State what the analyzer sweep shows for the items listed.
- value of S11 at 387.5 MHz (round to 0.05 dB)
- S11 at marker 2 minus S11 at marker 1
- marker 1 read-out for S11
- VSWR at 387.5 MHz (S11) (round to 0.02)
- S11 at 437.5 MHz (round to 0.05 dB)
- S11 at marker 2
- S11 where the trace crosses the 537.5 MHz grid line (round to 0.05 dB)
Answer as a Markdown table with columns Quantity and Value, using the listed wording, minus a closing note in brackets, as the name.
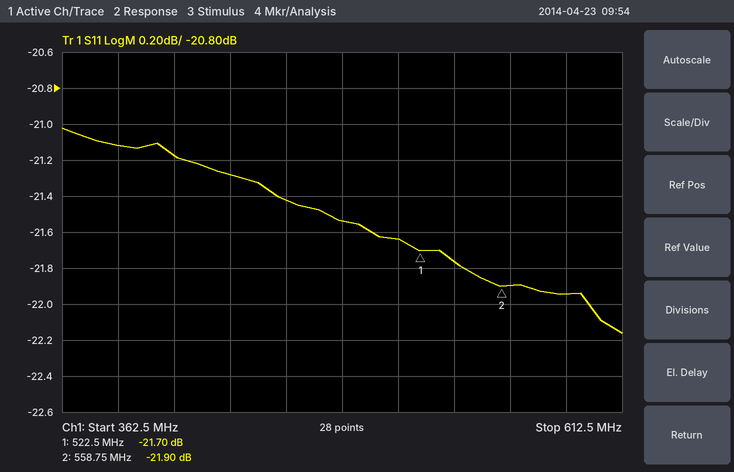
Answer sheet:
| Quantity | Value |
|---|---|
| value of S11 at 387.5 MHz | -21.10 dB |
| S11 at marker 2 minus S11 at marker 1 | -0.20 dB |
| marker 1 read-out for S11 | -21.70 dB |
| VSWR at 387.5 MHz (S11) | 1.20 |
| S11 at 437.5 MHz | -21.30 dB |
| S11 at marker 2 | -21.90 dB |
| S11 where the trace crosses the 537.5 MHz grid line | -21.75 dB |
